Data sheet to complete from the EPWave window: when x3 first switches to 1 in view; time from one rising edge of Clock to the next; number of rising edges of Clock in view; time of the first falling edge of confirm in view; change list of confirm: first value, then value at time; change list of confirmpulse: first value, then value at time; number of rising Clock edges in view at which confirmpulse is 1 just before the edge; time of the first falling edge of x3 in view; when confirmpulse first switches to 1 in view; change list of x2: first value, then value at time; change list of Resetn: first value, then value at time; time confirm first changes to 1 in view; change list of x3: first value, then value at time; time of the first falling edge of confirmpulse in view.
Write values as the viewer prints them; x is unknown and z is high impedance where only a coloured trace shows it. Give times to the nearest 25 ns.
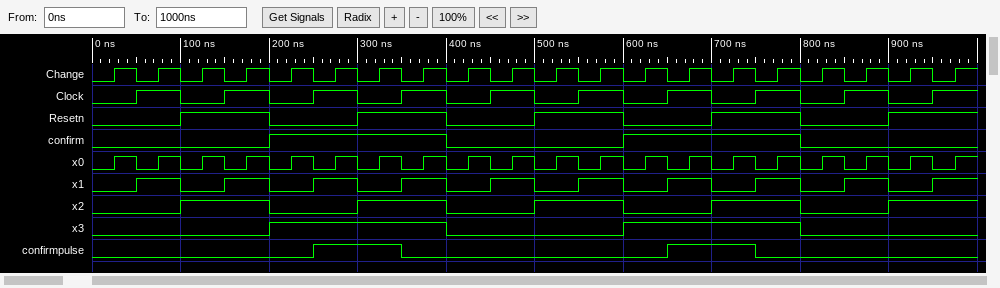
200 ns
100 ns
10
400 ns
0, 1 at 200 ns, 0 at 400 ns, 1 at 600 ns, 0 at 800 ns
0, 1 at 250 ns, 0 at 350 ns, 1 at 650 ns, 0 at 750 ns
2
400 ns
250 ns
0, 1 at 100 ns, 0 at 200 ns, 1 at 300 ns, 0 at 400 ns, 1 at 500 ns, 0 at 600 ns, 1 at 700 ns, 0 at 800 ns, 1 at 900 ns
0, 1 at 100 ns, 0 at 200 ns, 1 at 300 ns, 0 at 400 ns, 1 at 500 ns, 0 at 600 ns, 1 at 700 ns, 0 at 800 ns, 1 at 900 ns
200 ns
0, 1 at 200 ns, 0 at 400 ns, 1 at 600 ns, 0 at 800 ns
350 ns
